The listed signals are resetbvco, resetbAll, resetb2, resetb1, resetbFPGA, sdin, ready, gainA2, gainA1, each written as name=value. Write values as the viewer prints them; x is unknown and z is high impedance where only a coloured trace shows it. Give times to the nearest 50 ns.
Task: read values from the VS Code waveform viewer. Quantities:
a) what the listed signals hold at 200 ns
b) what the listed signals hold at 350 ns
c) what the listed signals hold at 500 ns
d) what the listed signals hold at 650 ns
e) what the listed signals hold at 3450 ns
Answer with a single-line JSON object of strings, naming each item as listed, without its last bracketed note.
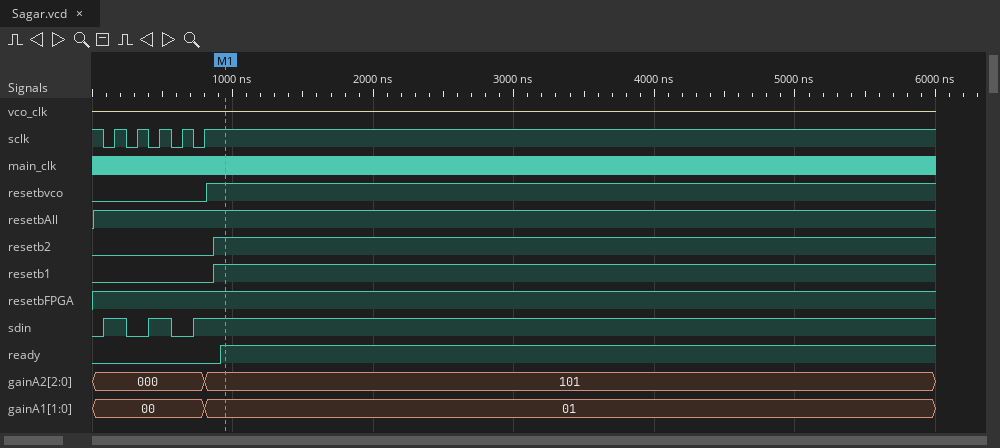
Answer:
{"what the listed signals hold at 200 ns": "resetbvco=0, resetbAll=1, resetb2=0, resetb1=0, resetbFPGA=1, sdin=1, ready=0, gainA2=000, gainA1=00", "what the listed signals hold at 350 ns": "resetbvco=0, resetbAll=1, resetb2=0, resetb1=0, resetbFPGA=1, sdin=0, ready=0, gainA2=000, gainA1=00", "what the listed signals hold at 500 ns": "resetbvco=0, resetbAll=1, resetb2=0, resetb1=0, resetbFPGA=1, sdin=1, ready=0, gainA2=000, gainA1=00", "what the listed signals hold at 650 ns": "resetbvco=0, resetbAll=1, resetb2=0, resetb1=0, resetbFPGA=1, sdin=0, ready=0, gainA2=000, gainA1=00", "what the listed signals hold at 3450 ns": "resetbvco=1, resetbAll=1, resetb2=1, resetb1=1, resetbFPGA=1, sdin=1, ready=1, gainA2=101, gainA1=01"}
